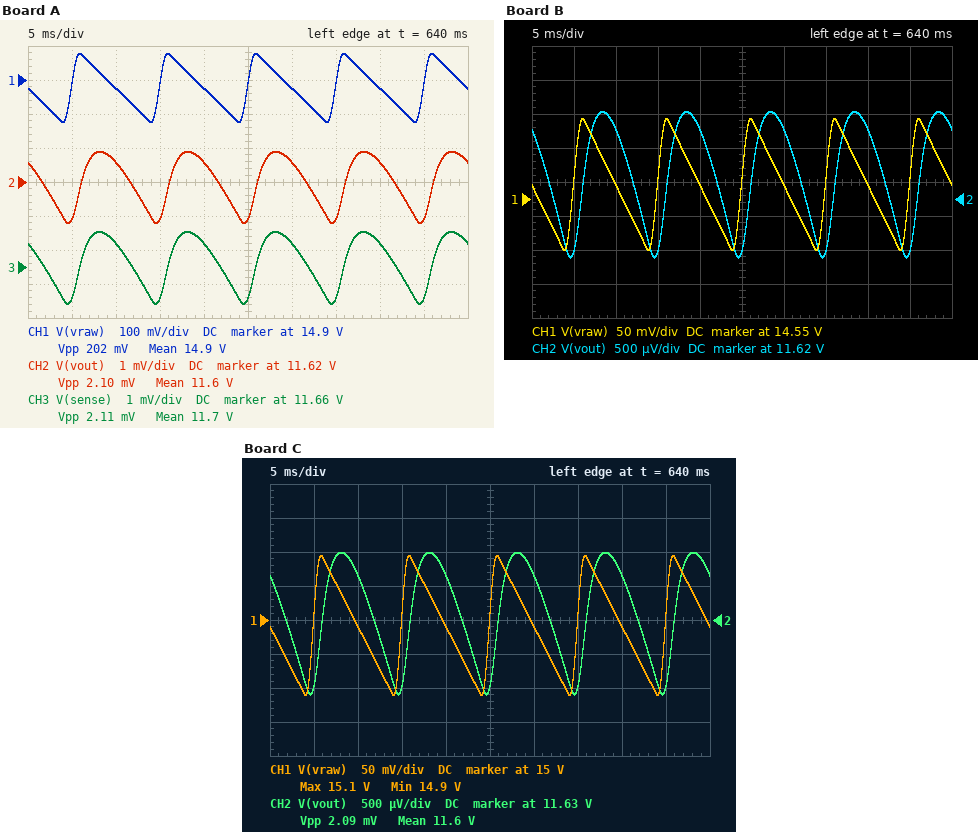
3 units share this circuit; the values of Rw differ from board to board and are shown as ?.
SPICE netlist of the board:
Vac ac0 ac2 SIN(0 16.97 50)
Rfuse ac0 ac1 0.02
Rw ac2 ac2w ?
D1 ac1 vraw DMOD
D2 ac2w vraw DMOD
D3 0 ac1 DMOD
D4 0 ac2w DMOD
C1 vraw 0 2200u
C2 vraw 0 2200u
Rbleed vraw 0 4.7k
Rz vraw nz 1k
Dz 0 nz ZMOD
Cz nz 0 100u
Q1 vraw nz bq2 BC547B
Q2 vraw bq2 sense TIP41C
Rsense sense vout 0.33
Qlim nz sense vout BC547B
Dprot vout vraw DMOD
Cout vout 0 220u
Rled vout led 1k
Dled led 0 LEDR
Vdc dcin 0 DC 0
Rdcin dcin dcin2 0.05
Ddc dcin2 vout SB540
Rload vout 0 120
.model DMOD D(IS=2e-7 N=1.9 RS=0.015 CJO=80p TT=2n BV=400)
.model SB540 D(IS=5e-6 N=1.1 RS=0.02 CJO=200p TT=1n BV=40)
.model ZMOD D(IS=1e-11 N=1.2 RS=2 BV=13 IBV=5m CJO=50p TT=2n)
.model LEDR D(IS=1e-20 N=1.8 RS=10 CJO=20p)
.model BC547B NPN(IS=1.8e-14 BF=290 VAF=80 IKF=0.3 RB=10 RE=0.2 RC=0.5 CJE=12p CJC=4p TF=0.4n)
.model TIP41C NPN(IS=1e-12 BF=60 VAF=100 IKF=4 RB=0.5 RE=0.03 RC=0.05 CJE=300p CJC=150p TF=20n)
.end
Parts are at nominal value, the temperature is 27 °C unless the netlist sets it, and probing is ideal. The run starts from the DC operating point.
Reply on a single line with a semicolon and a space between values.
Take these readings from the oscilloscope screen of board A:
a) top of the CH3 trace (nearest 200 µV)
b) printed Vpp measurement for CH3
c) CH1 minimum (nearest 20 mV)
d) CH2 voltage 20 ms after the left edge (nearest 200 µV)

11.6600 V; 2.11 mV; 14.78 V; 11.6246 V
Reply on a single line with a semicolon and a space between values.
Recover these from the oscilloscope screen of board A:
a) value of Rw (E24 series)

0.62 Ω
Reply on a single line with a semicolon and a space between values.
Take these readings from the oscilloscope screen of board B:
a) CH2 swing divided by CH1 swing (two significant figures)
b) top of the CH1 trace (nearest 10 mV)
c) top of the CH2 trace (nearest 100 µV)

0.011; 14.67 V; 11.6188 V
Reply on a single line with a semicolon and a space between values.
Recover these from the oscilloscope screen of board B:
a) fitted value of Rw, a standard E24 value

1.2 Ω
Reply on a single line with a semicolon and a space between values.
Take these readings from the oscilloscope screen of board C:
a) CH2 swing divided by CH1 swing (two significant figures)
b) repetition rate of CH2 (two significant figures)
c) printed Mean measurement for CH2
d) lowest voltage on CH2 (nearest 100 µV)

0.010; 100 Hz; 11.6 V; 11.6249 V
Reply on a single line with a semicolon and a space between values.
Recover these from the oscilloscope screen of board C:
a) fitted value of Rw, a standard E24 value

0.43 Ω
